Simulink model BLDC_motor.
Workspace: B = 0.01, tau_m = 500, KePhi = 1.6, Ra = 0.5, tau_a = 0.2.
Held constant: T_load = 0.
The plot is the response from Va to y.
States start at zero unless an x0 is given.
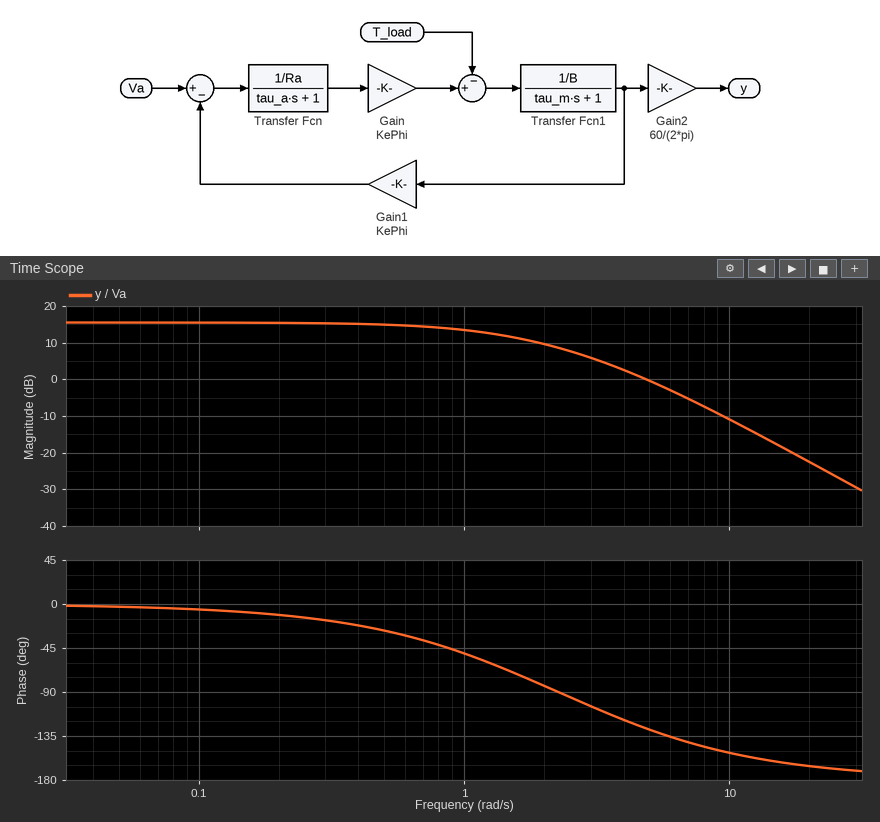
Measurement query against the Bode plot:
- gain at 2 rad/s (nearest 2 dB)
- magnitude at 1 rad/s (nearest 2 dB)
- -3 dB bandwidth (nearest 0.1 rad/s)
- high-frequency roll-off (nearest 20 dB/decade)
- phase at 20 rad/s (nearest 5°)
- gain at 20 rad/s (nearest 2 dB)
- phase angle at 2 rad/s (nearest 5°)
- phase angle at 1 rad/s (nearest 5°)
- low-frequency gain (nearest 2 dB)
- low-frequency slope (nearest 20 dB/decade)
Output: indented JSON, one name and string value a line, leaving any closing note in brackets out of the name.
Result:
{
  "gain at 2 rad/s": "10 dB",
  "magnitude at 1 rad/s": "14 dB",
  "-3 dB bandwidth": "1.3 rad/s",
  "high-frequency roll-off": "-40 dB/decade",
  "phase at 20 rad/s": "-165°",
  "gain at 20 rad/s": "-22 dB",
  "phase angle at 2 rad/s": "-85°",
  "phase angle at 1 rad/s": "-50°",
  "low-frequency gain": "16 dB",
  "low-frequency slope": "0 dB/decade"
}
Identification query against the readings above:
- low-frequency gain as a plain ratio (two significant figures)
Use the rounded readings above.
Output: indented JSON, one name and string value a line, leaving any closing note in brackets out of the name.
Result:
{
  "low-frequency gain as a plain ratio": "6.3"
}
